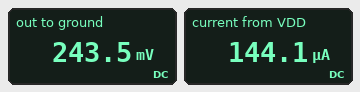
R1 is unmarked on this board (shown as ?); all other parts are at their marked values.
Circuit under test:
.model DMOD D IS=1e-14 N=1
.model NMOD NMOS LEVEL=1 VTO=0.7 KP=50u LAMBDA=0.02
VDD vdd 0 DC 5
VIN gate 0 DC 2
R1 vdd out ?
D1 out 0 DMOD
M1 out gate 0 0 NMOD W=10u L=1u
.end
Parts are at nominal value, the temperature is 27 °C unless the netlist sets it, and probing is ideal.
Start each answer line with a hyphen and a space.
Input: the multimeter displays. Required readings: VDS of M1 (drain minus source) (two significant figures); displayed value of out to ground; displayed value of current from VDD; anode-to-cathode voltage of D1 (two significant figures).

- 240 mV
- 243.5 mV
- 144.1 µA
- 240 mV
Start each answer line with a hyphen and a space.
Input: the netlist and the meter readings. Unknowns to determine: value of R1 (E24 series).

- 33 kΩ
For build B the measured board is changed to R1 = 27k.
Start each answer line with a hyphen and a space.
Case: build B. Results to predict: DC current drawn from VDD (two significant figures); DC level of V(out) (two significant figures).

- 170 µA
- 300 mV
